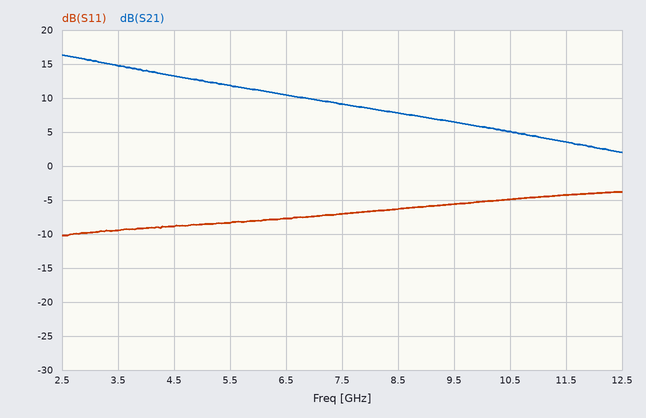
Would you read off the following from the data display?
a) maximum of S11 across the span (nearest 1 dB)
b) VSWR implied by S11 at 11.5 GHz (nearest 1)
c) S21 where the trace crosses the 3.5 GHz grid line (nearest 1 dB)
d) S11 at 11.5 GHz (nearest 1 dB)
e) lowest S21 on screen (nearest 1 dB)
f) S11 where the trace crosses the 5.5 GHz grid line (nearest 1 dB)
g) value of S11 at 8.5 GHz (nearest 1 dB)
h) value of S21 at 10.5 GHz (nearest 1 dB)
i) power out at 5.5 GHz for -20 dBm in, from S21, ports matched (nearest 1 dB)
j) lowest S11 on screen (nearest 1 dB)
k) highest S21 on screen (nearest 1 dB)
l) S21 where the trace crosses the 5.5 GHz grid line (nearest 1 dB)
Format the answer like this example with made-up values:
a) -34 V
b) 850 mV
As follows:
a) -4 dB
b) 4
c) 15 dB
d) -4 dB
e) 2 dB
f) -8 dB
g) -6 dB
h) 5 dB
i) -8 dBm
j) -10 dB
k) 16 dB
l) 12 dB
